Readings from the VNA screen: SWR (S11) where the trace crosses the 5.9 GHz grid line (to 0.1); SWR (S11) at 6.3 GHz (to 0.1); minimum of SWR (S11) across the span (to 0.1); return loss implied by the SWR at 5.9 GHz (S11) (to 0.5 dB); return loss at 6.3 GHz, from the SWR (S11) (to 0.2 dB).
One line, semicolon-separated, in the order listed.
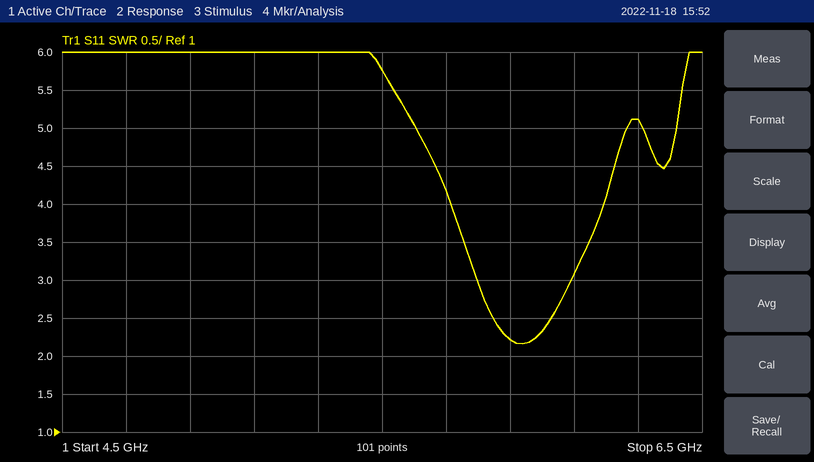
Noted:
2.2; 5.1; 2.2; 8.5 dB; 3.4 dB
